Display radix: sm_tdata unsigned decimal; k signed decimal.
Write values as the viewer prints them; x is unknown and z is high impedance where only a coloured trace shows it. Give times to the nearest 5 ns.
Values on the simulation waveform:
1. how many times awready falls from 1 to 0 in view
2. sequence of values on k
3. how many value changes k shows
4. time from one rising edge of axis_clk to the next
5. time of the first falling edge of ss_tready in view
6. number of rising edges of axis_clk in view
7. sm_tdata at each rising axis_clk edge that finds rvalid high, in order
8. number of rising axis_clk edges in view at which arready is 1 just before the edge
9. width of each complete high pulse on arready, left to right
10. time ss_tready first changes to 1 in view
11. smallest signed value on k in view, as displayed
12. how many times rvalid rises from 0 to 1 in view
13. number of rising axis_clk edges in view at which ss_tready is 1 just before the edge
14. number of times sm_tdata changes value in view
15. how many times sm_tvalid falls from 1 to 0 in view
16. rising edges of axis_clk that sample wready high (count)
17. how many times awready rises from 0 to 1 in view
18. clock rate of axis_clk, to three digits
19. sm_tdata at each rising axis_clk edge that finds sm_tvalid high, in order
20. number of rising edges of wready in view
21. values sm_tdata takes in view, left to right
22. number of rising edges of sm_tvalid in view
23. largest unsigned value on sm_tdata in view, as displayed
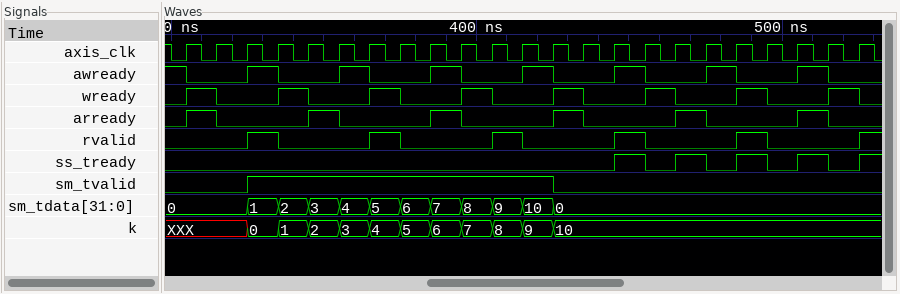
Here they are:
8
XXX, 0, 1, 2, 3, 4, 5, 6, 7, 8, 9, 10
11
10 ns
455 ns
23
1, 5, 9, 0, 0
6
10 ns, 10 ns, 10 ns, 10 ns, 10 ns, 10 ns
445 ns
0
6
4
11
1
8
7
100 MHz
1, 2, 3, 4, 5, 6, 7, 8, 9, 10
8
0, 1, 2, 3, 4, 5, 6, 7, 8, 9, 10, 0
1
10
